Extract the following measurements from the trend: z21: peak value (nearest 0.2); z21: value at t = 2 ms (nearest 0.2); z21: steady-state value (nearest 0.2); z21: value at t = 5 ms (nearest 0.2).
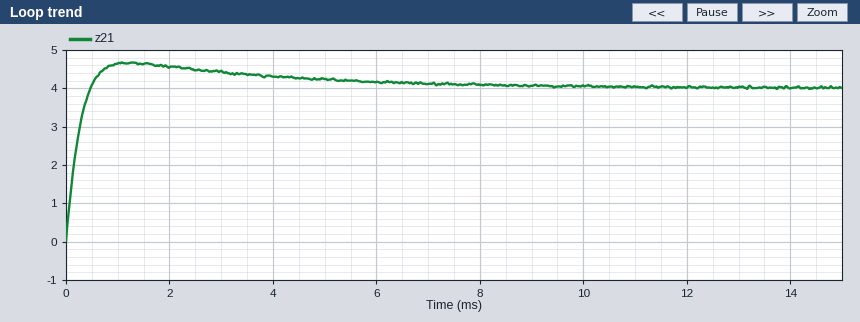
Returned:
4.6
4.6
4.0
4.2
